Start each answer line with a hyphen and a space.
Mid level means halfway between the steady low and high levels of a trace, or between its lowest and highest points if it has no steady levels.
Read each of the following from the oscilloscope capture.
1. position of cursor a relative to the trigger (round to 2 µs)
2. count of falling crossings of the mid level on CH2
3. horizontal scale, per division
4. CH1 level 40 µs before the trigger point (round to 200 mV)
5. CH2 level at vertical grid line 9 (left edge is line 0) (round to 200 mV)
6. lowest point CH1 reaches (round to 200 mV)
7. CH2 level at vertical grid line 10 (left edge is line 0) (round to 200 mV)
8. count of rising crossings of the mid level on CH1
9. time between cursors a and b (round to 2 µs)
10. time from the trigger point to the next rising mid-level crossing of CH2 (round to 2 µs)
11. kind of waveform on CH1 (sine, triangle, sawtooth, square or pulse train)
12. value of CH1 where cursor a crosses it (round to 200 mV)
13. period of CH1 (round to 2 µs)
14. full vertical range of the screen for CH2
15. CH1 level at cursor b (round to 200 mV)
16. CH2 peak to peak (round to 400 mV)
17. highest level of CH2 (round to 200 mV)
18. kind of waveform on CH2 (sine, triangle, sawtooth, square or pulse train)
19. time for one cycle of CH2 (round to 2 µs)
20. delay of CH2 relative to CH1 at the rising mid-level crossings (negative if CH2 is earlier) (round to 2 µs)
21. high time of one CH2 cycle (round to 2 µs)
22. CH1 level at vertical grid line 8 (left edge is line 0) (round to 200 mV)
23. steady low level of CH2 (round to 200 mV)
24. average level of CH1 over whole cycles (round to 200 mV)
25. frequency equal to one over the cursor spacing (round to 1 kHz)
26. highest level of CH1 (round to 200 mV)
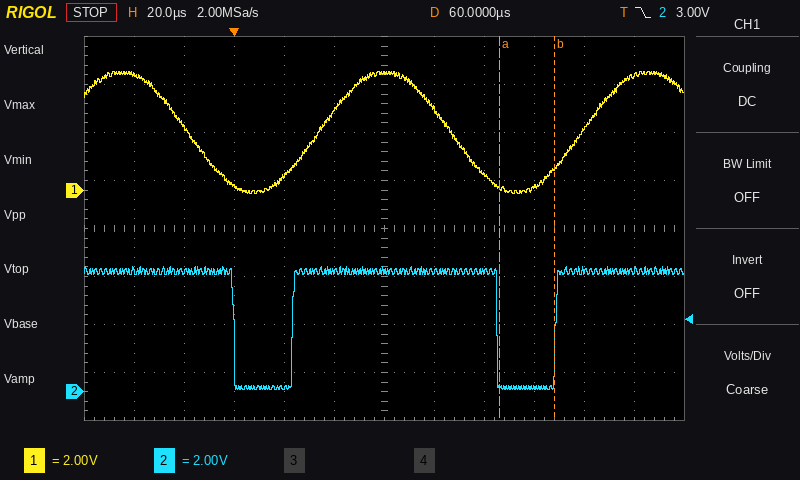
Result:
- +106 µs
- 2
- 20 µs
- 4.8 V
- 200 mV
- -200 mV
- 5.0 V
- 2
- 22 µs
- 24 µs
- sine
- 200 mV
- 106 µs
- 16 V
- 1.0 V
- 5.2 V
- 5.2 V
- pulse train
- 106 µs
- -10 µs
- 82 µs
- 600 mV
- 200 mV
- 2.4 V
- 45 kHz
- 5.0 V
